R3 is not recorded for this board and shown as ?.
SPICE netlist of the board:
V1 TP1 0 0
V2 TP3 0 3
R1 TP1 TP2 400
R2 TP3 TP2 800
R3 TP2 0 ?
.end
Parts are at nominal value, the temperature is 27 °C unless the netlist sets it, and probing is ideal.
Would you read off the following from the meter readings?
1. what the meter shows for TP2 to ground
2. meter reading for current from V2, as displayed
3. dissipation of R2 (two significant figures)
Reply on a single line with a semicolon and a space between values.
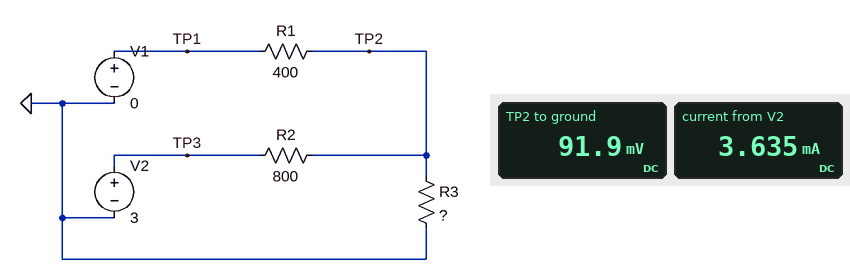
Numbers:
91.9 mV; 3.635 mA; 11 mW
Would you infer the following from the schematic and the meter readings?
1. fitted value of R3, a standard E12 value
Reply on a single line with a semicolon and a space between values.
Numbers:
27 Ω
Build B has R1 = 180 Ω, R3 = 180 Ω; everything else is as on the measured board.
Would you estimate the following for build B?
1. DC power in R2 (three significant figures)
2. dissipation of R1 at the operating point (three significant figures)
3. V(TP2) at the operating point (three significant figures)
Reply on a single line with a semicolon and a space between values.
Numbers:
9.09 mW; 511 µW; 303 mV
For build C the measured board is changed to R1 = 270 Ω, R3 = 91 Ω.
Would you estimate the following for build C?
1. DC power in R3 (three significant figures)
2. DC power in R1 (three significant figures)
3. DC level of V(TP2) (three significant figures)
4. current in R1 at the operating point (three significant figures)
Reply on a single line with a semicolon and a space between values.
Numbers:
608 µW; 205 µW; 235 mV; 871 µA
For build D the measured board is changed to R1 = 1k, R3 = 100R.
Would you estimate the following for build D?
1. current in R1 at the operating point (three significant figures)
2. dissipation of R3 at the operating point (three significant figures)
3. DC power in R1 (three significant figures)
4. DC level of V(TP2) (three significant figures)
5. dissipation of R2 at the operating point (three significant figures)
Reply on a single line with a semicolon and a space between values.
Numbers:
306 µA; 937 µW; 93.7 µW; 306 mV; 9.07 mW
